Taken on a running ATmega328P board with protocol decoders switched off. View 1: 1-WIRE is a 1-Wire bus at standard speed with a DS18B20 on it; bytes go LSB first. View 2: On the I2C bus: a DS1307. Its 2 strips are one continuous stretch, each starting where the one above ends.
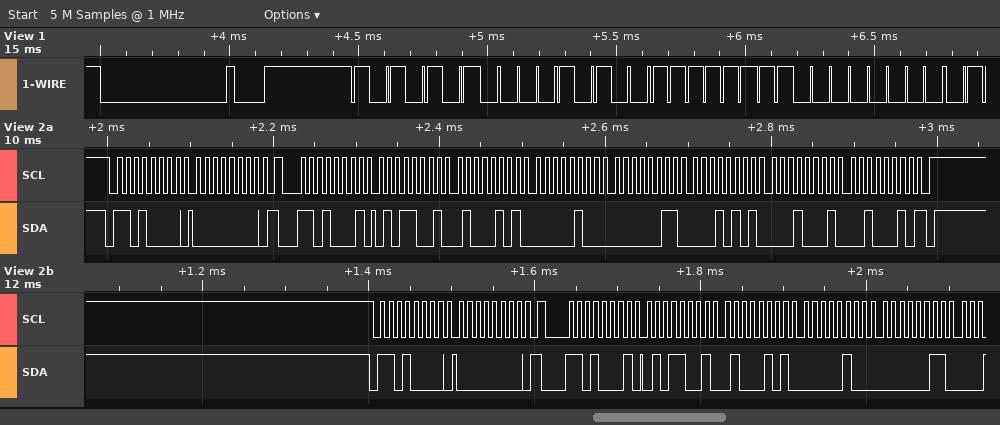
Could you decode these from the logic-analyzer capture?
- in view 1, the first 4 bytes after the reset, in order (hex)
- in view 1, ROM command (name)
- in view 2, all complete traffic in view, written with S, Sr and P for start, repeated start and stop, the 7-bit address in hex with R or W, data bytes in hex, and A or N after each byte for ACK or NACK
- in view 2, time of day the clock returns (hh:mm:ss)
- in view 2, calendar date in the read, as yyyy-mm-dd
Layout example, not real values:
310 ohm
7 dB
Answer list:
55 28 FF 00
Match ROM
S 68W A 00 A Sr 68R A 59 A 45 A 04 A 03 A 15 A 11 A 22 N P S 68W A 00 A Sr 68R A 59 A 45 A 04 A 03 A
04:45:59
2022-11-15
